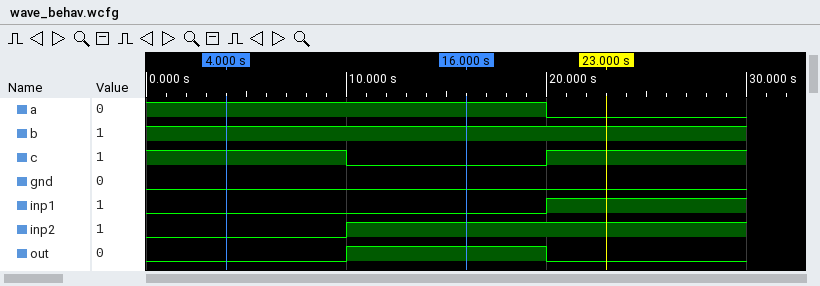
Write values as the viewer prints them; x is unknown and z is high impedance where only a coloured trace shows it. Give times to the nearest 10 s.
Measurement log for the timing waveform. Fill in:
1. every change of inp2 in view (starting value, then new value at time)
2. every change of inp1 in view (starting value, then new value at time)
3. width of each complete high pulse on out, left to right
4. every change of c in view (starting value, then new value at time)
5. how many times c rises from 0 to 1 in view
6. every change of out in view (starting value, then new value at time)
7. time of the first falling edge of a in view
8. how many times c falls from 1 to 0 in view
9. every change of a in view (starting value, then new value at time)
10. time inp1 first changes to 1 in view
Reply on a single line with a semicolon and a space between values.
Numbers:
0, 1 at 10 s; 0, 1 at 20 s; 10 s; 1, 0 at 10 s, 1 at 20 s; 1; 0, 1 at 10 s, 0 at 20 s; 20 s; 1; 1, 0 at 20 s; 20 s
